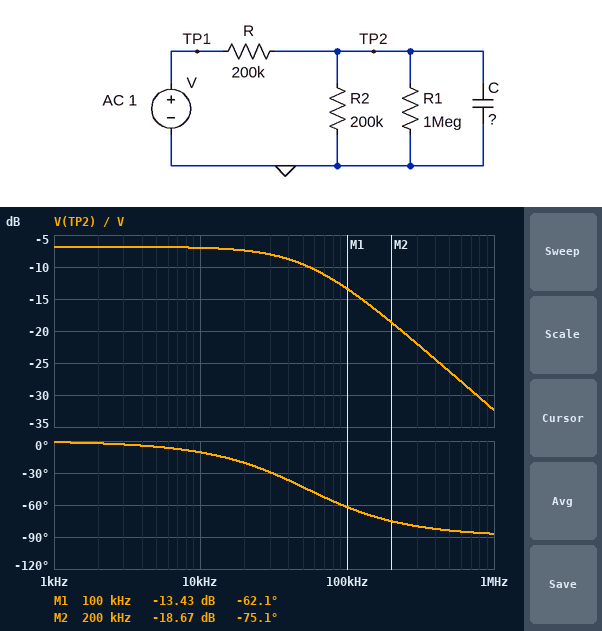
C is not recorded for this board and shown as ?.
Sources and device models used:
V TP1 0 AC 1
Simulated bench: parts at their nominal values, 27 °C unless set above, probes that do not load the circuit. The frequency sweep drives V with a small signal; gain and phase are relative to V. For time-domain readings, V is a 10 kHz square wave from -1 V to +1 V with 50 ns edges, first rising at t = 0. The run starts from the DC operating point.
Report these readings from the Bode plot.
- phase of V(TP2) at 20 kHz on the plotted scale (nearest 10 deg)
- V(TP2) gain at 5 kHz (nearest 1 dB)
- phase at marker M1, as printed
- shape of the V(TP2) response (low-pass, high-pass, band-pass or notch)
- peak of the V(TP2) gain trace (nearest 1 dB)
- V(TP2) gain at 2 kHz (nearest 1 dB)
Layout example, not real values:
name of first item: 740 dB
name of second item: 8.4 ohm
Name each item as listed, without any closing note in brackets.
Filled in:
phase of V(TP2) at 20 kHz on the plotted scale: -20 deg
V(TP2) gain at 5 kHz: -7 dB
phase at marker M1, as printed: -62.1 deg
shape of the V(TP2) response: low-pass
peak of the V(TP2) gain trace: -7 dB
V(TP2) gain at 2 kHz: -7 dB
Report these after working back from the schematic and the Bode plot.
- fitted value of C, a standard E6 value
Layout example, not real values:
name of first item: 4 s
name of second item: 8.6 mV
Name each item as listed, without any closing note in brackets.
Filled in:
fitted value of C, a standard E6 value: 33 pF
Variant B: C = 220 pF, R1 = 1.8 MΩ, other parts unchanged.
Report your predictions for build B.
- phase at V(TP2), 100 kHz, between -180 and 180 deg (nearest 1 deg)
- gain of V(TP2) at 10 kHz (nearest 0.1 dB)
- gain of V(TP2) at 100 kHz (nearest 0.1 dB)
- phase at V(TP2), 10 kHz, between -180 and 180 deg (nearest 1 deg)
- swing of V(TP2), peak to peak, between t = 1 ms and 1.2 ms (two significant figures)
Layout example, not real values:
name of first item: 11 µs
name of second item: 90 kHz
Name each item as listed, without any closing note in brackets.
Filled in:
phase at V(TP2), 100 kHz, between -180 and 180 deg: -86 deg
gain of V(TP2) at 10 kHz: -10.8 dB
gain of V(TP2) at 100 kHz: -28.9 dB
phase at V(TP2), 10 kHz, between -180 and 180 deg: -53 deg
swing of V(TP2), peak to peak, between t = 1 ms and 1.2 ms: 790 mV
